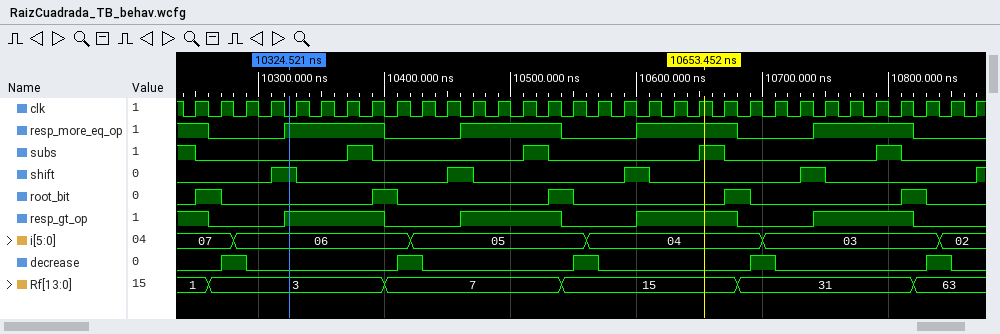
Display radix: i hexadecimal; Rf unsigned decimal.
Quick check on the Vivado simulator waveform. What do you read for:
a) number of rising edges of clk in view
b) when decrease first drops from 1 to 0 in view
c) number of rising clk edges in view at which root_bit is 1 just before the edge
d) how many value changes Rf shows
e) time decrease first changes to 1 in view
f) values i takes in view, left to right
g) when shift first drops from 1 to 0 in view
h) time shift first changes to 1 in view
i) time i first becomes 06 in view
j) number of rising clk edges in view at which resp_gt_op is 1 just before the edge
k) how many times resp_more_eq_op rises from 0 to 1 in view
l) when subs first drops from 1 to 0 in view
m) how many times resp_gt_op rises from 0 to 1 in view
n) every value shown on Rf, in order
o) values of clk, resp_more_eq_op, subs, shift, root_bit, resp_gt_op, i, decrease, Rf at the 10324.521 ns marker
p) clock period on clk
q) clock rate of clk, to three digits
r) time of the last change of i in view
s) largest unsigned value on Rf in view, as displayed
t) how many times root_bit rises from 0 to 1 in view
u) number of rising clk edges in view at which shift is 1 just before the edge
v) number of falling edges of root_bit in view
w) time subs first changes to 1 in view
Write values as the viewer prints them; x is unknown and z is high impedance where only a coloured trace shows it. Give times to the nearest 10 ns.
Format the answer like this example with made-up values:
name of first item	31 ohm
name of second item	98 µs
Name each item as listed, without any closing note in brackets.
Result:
number of rising edges of clk in view	32
when decrease first drops from 1 to 0 in view	10290 ns
number of rising clk edges in view at which root_bit is 1 just before the edge	5
how many value changes Rf shows	5
time decrease first changes to 1 in view	10270 ns
values i takes in view, left to right	07, 06, 05, 04, 03, 02
when shift first drops from 1 to 0 in view	10330 ns
time shift first changes to 1 in view	10310 ns
time i first becomes 06 in view	10280 ns
number of rising clk edges in view at which resp_gt_op is 1 just before the edge	17
how many times resp_more_eq_op rises from 0 to 1 in view	4
when subs first drops from 1 to 0 in view	10250 ns
how many times resp_gt_op rises from 0 to 1 in view	4
every value shown on Rf, in order	1, 3, 7, 15, 31, 63
values of clk, resp_more_eq_op, subs, shift, root_bit, resp_gt_op, i, decrease, Rf at the 10324.521 ns marker	clk=0, resp_more_eq_op=1, subs=0, shift=1, root_bit=0, resp_gt_op=1, i=06, decrease=0, Rf=3
clock period on clk	20 ns
clock rate of clk, to three digits	50.0 MHz
time of the last change of i in view	10840 ns
largest unsigned value on Rf in view, as displayed	63
how many times root_bit rises from 0 to 1 in view	5
number of rising clk edges in view at which shift is 1 just before the edge	4
number of falling edges of root_bit in view	5
time subs first changes to 1 in view	10370 ns
